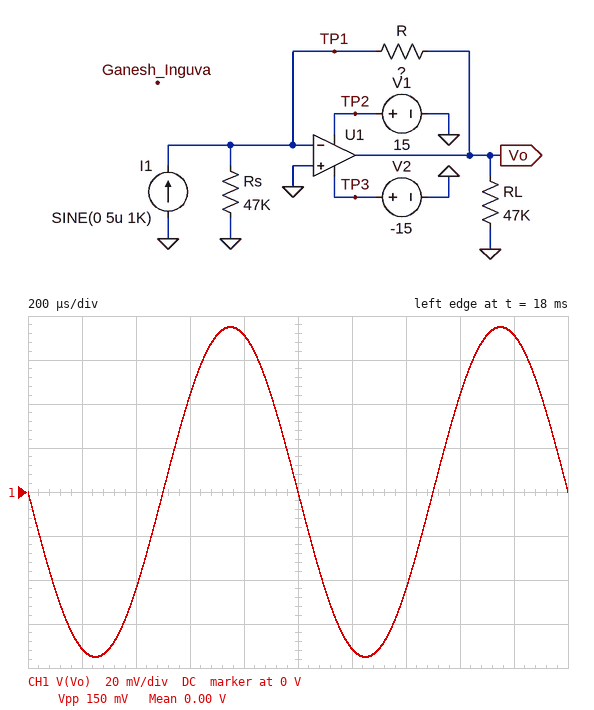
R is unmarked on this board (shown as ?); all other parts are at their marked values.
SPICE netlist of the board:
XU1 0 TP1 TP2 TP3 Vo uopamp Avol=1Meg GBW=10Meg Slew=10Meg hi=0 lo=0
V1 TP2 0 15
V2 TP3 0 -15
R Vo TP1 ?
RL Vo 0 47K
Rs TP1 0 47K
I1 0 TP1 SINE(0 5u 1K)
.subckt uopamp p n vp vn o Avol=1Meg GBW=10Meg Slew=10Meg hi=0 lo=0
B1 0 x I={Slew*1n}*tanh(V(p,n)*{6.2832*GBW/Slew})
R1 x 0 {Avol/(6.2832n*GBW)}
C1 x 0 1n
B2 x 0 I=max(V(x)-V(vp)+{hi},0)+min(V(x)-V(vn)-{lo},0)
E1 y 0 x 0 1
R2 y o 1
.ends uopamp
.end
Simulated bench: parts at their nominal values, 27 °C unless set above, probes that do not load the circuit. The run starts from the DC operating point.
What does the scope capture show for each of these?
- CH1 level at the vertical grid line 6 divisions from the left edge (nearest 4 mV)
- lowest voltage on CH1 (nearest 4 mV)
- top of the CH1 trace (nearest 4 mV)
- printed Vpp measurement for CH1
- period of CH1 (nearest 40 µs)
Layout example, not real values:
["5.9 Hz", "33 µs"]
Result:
["-72 mV", "-76 mV", "76 mV", "150 mV", "1.00 ms"]
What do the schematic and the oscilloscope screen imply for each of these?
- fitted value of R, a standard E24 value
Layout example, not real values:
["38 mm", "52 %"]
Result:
["15 kΩ"]
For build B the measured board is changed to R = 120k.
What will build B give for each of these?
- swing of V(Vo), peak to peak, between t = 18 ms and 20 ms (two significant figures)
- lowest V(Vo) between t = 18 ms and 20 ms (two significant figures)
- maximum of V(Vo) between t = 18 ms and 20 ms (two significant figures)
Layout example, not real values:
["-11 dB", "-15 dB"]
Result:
["1.2 V", "-600 mV", "600 mV"]
